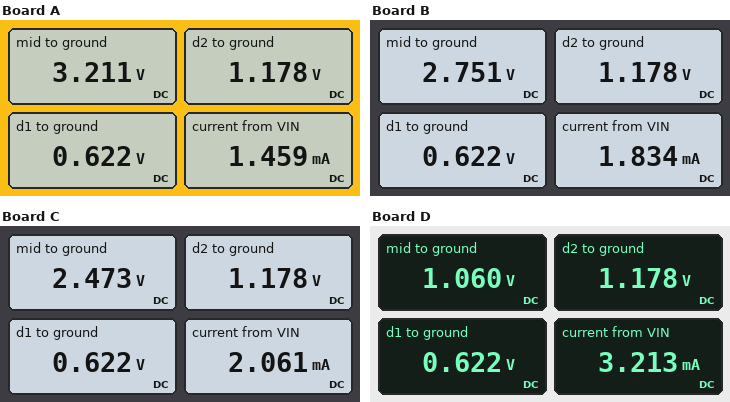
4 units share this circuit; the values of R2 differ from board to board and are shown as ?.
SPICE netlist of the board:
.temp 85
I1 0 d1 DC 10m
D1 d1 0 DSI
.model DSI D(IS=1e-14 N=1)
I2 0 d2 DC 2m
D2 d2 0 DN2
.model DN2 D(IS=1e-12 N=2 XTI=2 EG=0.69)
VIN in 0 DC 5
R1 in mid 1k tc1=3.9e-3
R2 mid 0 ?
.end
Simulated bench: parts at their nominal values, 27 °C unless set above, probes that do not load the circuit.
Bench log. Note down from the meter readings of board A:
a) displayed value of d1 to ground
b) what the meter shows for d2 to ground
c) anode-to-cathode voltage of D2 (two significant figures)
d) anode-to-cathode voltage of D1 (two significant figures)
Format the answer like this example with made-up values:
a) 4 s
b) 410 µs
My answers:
a) 0.622 V
b) 1.178 V
c) 1.2 V
d) 620 mV
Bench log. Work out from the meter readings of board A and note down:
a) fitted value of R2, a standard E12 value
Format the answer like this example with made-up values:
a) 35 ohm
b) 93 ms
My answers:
a) 2.2 kΩ
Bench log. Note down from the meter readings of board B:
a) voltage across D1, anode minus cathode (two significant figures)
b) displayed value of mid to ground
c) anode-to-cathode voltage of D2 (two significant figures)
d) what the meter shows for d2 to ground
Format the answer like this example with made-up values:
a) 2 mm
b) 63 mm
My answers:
a) 620 mV
b) 2.751 V
c) 1.2 V
d) 1.178 V
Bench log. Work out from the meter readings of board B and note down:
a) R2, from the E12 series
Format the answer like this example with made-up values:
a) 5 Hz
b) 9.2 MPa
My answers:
a) 1.5 kΩ
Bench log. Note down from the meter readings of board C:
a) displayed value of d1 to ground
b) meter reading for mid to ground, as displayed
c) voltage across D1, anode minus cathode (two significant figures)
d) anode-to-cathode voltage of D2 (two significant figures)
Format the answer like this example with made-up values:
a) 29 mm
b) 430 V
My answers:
a) 0.622 V
b) 2.473 V
c) 620 mV
d) 1.2 V
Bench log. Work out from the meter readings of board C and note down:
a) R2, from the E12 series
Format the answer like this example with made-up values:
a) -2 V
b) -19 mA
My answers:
a) 1.2 kΩ
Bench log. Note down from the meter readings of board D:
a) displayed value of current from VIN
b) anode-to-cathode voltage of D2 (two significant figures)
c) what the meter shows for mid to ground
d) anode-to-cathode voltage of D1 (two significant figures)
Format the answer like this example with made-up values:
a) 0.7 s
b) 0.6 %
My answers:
a) 3.213 mA
b) 1.2 V
c) 1.060 V
d) 620 mV
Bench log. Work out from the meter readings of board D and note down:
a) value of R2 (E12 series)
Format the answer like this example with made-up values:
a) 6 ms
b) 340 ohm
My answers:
a) 330 Ω
